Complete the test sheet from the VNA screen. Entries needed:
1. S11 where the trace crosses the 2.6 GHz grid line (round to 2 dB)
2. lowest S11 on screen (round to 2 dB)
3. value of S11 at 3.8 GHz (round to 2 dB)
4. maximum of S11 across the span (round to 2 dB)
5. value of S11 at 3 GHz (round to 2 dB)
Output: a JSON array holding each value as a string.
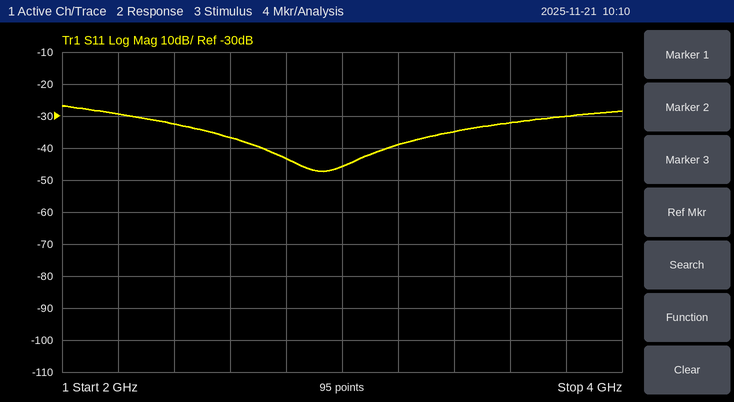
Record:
["-36 dB", "-48 dB", "-30 dB", "-26 dB", "-46 dB"]
